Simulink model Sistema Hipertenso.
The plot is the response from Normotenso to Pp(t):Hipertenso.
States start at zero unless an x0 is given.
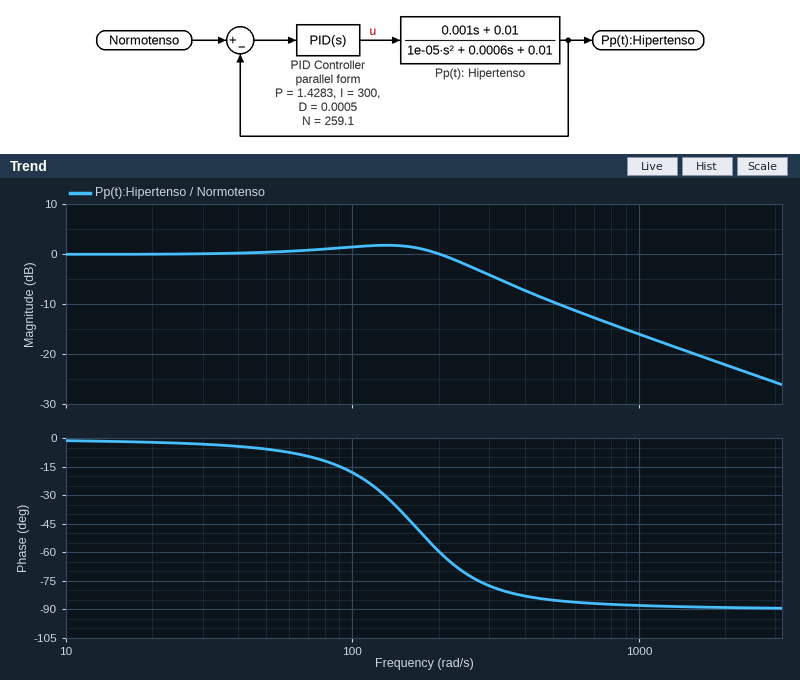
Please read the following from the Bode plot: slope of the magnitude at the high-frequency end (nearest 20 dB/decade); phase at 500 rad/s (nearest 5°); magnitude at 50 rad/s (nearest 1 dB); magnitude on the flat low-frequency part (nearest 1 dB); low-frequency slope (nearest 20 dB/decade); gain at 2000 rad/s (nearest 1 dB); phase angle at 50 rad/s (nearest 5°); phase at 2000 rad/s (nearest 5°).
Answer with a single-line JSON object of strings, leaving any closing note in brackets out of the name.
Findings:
{"slope of the magnitude at the high-frequency end": "-20 dB/decade", "phase at 500 rad/s": "-85°", "magnitude at 50 rad/s": "0 dB", "magnitude on the flat low-frequency part": "0 dB", "low-frequency slope": "0 dB/decade", "gain at 2000 rad/s": "-22 dB", "phase angle at 50 rad/s": "-5°", "phase at 2000 rad/s": "-90°"}
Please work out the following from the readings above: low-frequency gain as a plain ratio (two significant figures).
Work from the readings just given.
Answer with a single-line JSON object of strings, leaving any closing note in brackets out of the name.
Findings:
{"low-frequency gain as a plain ratio": "1.0"}
